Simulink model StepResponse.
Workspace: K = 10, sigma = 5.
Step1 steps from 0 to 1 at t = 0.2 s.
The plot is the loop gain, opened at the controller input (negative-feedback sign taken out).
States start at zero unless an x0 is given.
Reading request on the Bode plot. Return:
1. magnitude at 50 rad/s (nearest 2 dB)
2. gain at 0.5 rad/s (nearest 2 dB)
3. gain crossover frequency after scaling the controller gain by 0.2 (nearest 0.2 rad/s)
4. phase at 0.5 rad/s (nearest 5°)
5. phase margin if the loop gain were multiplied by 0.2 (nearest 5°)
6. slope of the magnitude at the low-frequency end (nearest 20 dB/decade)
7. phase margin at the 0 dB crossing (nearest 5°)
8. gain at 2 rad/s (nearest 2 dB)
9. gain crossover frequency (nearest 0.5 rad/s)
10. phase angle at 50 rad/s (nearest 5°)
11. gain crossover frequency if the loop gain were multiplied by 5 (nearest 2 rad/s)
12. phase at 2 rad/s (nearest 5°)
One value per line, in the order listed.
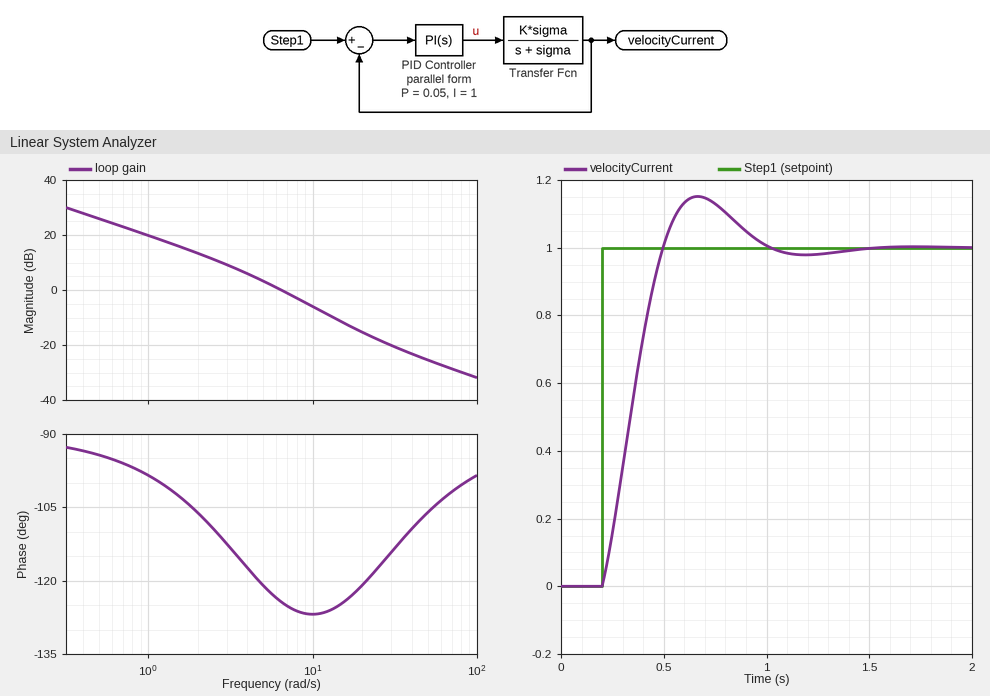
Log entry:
-26 dB
26 dB
1.8 rad/s
-95°
75°
-20 dB/decade
55°
14 dB
6.5 rad/s
-105°
18 rad/s
-105°
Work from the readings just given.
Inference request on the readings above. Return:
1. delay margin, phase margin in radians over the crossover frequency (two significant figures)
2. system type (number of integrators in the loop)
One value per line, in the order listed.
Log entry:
0.15 s
1
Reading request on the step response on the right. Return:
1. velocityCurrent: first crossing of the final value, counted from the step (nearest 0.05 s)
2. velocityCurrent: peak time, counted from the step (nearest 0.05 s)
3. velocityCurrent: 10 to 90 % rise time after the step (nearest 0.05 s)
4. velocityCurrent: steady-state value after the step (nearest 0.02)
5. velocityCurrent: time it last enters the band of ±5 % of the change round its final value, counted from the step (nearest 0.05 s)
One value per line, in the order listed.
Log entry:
0.30 s
0.45 s
0.20 s
1.00
0.70 s
